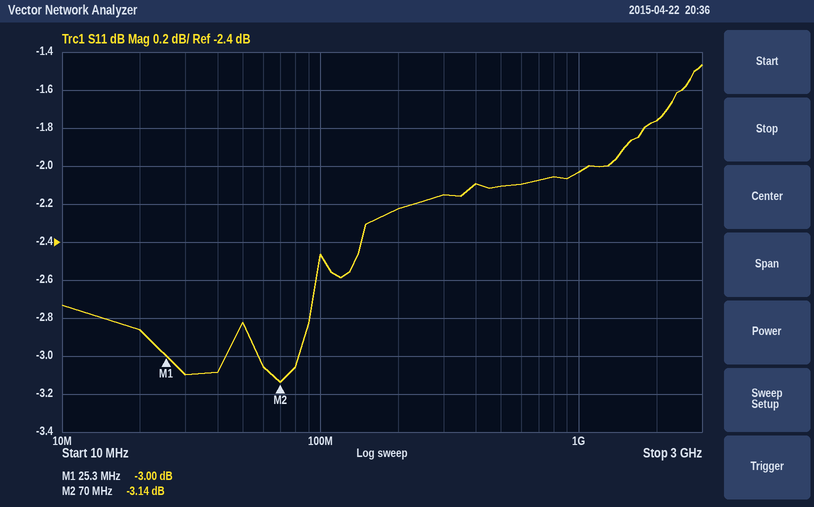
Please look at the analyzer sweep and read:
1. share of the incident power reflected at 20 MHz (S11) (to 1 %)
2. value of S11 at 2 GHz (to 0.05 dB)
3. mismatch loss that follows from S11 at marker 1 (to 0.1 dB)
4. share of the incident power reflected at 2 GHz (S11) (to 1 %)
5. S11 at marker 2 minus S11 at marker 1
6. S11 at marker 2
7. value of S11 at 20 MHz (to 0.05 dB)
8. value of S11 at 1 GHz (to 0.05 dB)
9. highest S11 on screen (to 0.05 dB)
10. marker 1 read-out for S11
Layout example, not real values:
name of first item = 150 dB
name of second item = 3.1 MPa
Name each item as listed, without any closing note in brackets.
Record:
share of the incident power reflected at 20 MHz (S11) = 52 %
value of S11 at 2 GHz = -1.75 dB
mismatch loss that follows from S11 at marker 1 = 3.0 dB
share of the incident power reflected at 2 GHz (S11) = 67 %
S11 at marker 2 minus S11 at marker 1 = -0.14 dB
S11 at marker 2 = -3.14 dB
value of S11 at 20 MHz = -2.85 dB
value of S11 at 1 GHz = -2.05 dB
highest S11 on screen = -1.45 dB
marker 1 read-out for S11 = -3.00 dB
